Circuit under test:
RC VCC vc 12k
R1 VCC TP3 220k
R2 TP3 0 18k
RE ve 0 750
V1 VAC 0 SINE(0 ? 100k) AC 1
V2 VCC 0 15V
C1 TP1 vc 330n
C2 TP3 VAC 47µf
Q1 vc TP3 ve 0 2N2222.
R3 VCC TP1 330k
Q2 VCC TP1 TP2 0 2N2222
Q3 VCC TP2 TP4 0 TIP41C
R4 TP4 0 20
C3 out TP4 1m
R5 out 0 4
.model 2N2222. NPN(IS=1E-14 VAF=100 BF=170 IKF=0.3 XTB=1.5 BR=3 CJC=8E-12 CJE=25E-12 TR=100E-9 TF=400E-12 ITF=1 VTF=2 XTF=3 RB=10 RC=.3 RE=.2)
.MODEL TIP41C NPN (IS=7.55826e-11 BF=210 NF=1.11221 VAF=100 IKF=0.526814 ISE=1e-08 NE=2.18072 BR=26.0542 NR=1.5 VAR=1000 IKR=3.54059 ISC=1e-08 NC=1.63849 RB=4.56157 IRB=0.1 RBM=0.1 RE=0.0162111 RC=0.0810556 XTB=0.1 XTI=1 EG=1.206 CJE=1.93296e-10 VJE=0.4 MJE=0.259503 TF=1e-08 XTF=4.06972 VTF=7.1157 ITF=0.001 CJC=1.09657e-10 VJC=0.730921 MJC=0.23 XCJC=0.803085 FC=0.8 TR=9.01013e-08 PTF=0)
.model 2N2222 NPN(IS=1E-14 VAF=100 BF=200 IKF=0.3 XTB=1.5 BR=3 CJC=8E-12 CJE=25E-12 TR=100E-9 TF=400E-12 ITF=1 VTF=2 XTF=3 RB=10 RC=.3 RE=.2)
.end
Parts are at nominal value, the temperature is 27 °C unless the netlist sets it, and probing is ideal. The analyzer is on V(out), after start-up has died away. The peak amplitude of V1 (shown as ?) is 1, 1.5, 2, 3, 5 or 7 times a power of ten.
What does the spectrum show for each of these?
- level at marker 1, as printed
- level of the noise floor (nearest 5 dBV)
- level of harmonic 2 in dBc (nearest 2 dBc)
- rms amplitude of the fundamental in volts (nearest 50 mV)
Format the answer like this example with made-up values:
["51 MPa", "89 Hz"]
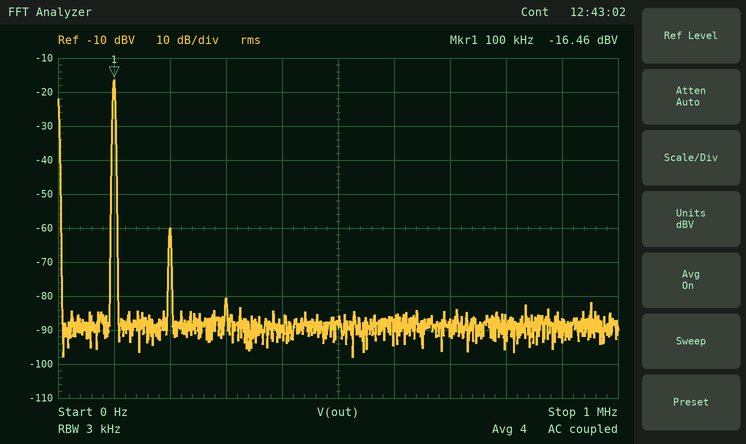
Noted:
["-16.46 dBV", "-90 dBV", "-44 dBc", "150 mV"]
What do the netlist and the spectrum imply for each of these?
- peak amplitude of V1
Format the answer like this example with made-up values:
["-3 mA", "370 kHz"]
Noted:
["20 mV"]
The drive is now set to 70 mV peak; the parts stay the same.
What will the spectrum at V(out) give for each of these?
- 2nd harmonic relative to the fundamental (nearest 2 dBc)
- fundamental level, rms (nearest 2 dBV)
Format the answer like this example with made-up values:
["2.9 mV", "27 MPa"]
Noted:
["-24 dBc", "-6 dBV"]
